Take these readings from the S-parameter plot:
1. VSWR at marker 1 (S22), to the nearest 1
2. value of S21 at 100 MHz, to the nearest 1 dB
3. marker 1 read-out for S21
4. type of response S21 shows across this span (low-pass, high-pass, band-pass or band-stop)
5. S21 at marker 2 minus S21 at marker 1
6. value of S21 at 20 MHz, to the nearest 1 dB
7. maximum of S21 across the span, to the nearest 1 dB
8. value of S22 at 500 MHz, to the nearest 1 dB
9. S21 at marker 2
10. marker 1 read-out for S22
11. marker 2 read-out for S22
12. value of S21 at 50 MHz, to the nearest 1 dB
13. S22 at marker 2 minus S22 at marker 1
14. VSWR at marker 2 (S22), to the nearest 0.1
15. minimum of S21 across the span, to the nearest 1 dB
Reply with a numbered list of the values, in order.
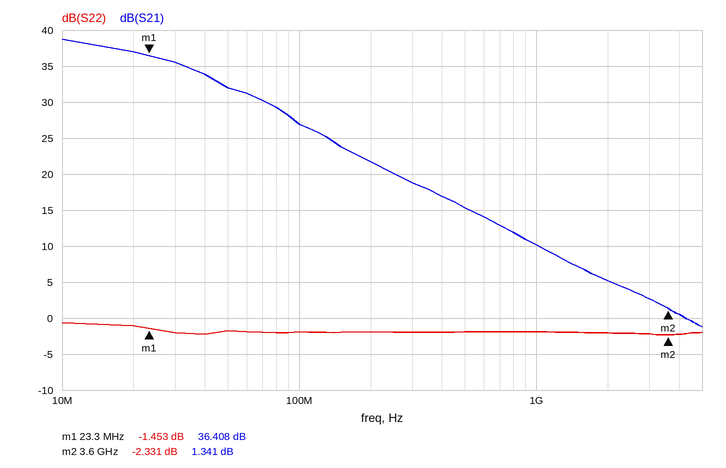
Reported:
1. 12
2. 27 dB
3. 36.408 dB
4. low-pass
5. -35.067 dB
6. 37 dB
7. 39 dB
8. -2 dB
9. 1.341 dB
10. -1.453 dB
11. -2.331 dB
12. 32 dB
13. -0.878 dB
14. 7.5
15. -1 dB
